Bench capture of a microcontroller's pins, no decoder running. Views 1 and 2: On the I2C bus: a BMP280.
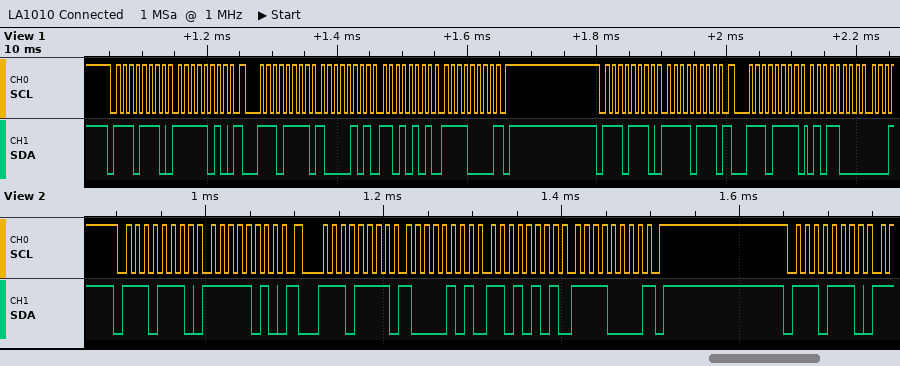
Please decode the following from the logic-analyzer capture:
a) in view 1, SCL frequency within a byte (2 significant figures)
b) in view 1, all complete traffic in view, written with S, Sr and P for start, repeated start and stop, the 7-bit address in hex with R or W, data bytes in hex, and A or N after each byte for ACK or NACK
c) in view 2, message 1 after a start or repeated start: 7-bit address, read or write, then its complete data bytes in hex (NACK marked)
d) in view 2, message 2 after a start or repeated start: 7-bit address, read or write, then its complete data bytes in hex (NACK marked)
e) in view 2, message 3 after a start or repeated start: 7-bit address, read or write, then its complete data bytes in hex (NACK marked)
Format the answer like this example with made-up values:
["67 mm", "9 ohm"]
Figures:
["100 kHz", "S 77W A FA A Sr 77R A 85 A D5 A F0 N P S 77W A F7 A Sr 77R A 58 A", "0x77 write: FA", "0x77 read: 85 D5 F0 NACK", "0x77 write"]
